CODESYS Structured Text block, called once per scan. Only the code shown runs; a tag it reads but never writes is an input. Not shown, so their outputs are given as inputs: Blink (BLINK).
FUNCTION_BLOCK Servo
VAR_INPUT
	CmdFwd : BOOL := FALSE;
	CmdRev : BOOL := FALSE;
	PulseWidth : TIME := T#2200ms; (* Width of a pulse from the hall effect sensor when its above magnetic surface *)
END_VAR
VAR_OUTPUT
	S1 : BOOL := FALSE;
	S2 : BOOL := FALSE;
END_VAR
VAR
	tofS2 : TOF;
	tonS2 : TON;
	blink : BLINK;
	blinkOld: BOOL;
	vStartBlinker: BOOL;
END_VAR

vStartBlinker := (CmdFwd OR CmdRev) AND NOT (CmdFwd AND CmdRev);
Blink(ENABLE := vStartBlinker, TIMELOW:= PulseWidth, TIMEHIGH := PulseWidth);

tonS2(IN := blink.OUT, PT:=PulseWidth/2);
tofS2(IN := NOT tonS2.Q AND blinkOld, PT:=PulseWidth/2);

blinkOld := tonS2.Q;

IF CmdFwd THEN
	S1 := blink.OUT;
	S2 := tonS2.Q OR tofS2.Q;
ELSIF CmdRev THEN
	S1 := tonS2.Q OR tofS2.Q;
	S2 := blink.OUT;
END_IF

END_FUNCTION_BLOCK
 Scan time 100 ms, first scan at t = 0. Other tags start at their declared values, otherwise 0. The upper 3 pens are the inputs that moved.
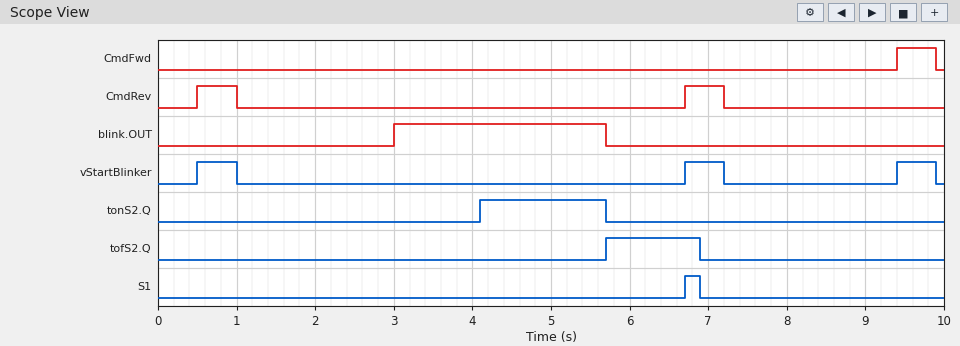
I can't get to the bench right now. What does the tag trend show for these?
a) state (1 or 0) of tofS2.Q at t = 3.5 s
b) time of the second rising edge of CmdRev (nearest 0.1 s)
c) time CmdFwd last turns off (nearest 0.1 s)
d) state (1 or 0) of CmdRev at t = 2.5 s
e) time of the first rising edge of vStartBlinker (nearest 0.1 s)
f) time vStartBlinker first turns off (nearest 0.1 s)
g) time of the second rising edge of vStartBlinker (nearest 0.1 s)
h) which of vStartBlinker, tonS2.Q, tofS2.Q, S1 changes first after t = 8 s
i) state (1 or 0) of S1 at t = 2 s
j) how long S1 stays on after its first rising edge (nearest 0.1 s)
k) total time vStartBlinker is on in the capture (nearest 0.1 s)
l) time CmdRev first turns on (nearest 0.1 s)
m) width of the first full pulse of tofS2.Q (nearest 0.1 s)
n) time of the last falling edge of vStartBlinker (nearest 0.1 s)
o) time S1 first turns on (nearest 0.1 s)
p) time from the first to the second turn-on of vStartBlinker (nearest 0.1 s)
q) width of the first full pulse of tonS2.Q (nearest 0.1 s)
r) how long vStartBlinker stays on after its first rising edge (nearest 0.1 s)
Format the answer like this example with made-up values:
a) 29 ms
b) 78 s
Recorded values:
a) 0
b) 6.7 s
c) 9.9 s
d) 0
e) 0.5 s
f) 1.0 s
g) 6.7 s
h) vStartBlinker
i) 0
j) 0.2 s
k) 1.5 s
l) 0.5 s
m) 1.2 s
n) 9.9 s
o) 6.7 s
p) 6.2 s
q) 1.6 s
r) 0.5 s
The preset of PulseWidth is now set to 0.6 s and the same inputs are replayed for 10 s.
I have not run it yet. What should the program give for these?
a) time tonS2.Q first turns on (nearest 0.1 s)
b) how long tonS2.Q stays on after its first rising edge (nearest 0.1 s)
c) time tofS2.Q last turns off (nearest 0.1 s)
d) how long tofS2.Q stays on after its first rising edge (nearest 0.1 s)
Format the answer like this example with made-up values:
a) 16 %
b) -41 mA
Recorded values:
a) 3.3 s
b) 2.4 s
c) 6.1 s
d) 0.4 s
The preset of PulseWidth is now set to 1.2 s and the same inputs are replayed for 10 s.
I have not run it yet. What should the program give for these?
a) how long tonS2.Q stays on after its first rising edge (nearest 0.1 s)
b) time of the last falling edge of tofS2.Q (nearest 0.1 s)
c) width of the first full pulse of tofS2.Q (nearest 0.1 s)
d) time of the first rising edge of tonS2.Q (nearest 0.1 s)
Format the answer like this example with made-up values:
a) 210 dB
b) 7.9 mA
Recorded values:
a) 2.1 s
b) 6.4 s
c) 0.7 s
d) 3.6 s
